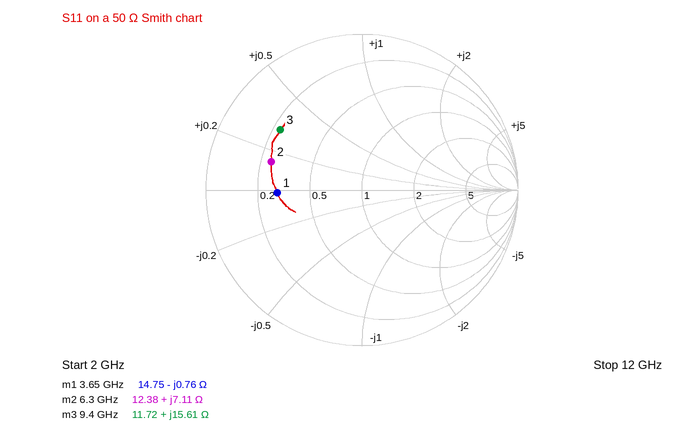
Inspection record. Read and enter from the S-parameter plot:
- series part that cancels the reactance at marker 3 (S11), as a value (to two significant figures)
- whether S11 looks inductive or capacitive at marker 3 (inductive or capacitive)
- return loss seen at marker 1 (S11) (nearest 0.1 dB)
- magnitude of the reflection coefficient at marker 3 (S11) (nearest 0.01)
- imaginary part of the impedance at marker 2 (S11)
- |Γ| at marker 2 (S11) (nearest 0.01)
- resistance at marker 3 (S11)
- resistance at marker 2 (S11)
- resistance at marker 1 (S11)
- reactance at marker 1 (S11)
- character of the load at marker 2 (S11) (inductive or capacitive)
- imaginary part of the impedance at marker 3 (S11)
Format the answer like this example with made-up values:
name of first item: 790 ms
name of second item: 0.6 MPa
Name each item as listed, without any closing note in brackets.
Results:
series part that cancels the reactance at marker 3 (S11), as a value: 1.1 pF
whether S11 looks inductive or capacitive at marker 3: inductive
return loss seen at marker 1 (S11): 5.3 dB
magnitude of the reflection coefficient at marker 3 (S11): 0.65
imaginary part of the impedance at marker 2: +7.11 Ω
|Γ| at marker 2 (S11): 0.61
resistance at marker 3: 11.72 Ω
resistance at marker 2: 12.38 Ω
resistance at marker 1: 14.75 Ω
reactance at marker 1: -0.76 Ω
character of the load at marker 2 (S11): inductive
imaginary part of the impedance at marker 3: +15.61 Ω
